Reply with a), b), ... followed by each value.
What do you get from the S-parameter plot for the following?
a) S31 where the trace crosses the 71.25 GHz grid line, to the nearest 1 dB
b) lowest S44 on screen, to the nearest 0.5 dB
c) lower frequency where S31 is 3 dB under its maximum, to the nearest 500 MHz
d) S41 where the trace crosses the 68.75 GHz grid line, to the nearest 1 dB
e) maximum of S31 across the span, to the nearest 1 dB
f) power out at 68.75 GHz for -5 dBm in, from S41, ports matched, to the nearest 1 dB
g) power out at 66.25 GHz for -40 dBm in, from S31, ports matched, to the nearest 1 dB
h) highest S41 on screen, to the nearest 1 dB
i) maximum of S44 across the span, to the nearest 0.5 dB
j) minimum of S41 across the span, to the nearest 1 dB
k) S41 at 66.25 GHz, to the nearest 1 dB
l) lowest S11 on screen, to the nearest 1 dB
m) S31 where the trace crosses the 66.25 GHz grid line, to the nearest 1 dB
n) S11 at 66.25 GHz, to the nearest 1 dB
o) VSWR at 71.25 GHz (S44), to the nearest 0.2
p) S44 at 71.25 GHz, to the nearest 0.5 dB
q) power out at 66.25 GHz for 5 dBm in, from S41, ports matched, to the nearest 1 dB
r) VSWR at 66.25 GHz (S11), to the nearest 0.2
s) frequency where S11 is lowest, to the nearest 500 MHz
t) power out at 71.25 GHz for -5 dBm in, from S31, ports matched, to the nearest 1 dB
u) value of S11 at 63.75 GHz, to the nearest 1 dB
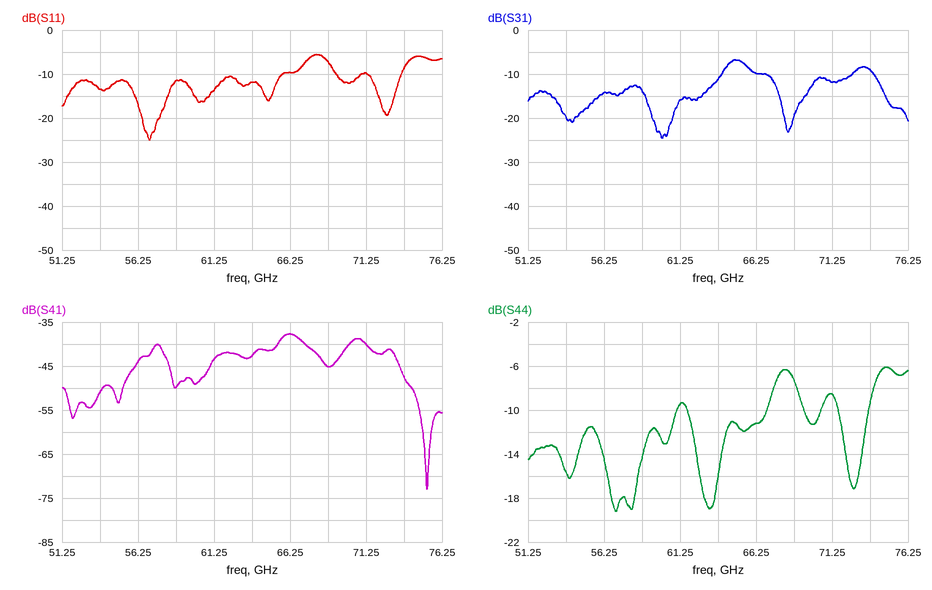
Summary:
a) -12 dB
b) -19.0 dB
c) 64.0 GHz
d) -45 dB
e) -7 dB
f) -50 dBm
g) -50 dBm
h) -38 dB
i) -6.0 dB
j) -73 dB
k) -38 dB
l) -25 dB
m) -10 dB
n) -10 dB
o) 2.2
p) -8.5 dB
q) -33 dBm
r) 2.0
s) 57.0 GHz
t) -17 dBm
u) -12 dB
